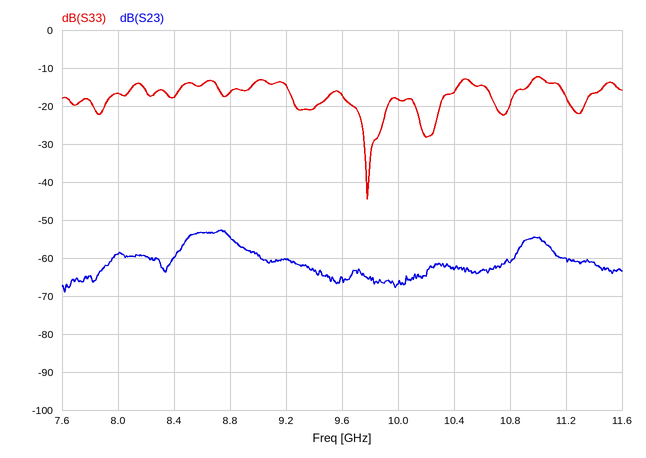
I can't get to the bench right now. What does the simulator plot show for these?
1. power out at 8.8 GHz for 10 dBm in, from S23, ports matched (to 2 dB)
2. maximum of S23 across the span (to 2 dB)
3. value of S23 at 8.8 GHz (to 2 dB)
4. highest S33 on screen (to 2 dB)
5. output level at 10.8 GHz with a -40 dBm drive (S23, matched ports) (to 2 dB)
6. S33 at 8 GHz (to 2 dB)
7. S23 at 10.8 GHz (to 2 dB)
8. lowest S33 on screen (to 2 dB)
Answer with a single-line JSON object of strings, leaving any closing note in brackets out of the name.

{"power out at 8.8 GHz for 10 dBm in, from S23, ports matched": "-44 dBm", "maximum of S23 across the span": "-52 dB", "value of S23 at 8.8 GHz": "-54 dB", "highest S33 on screen": "-12 dB", "output level at 10.8 GHz with a -40 dBm drive (S23, matched ports)": "-102 dBm", "S33 at 8 GHz": "-16 dB", "S23 at 10.8 GHz": "-62 dB", "lowest S33 on screen": "-44 dB"}
